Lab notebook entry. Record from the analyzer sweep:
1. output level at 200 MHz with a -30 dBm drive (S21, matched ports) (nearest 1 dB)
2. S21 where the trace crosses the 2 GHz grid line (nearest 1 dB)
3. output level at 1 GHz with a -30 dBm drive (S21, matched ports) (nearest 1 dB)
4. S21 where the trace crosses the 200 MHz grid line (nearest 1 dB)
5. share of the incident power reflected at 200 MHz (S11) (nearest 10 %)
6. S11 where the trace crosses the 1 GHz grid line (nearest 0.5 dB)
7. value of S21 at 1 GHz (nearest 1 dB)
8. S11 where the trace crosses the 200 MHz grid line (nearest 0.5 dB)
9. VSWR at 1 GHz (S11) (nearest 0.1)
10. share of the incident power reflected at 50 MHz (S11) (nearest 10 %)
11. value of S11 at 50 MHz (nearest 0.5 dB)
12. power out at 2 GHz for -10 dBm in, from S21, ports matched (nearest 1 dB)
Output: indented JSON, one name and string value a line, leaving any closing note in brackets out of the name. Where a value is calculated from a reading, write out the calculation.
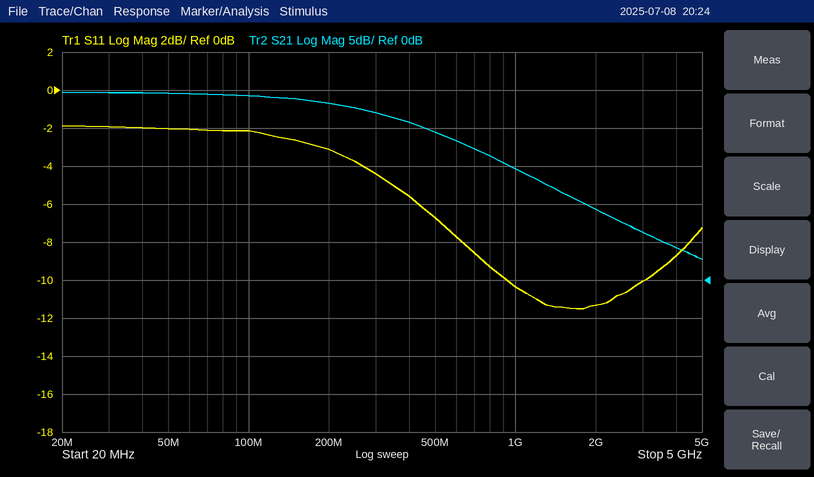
{
  "output level at 200 MHz with a -30 dBm drive (S21, matched ports)": "-30 dBm + (23 dB) = -7 dBm",
  "S21 where the trace crosses the 2 GHz grid line": "9 dB",
  "output level at 1 GHz with a -30 dBm drive (S21, matched ports)": "-30 dBm + (15 dB) = -15 dBm",
  "S21 where the trace crosses the 200 MHz grid line": "23 dB",
  "share of the incident power reflected at 200 MHz (S11)": "10^(-3/10) ≈ 50 %",
  "S11 where the trace crosses the 1 GHz grid line": "-10.5 dB",
  "value of S21 at 1 GHz": "15 dB",
  "S11 where the trace crosses the 200 MHz grid line": "-3.0 dB",
  "VSWR at 1 GHz (S11)": "|Γ| = 10^(-10.5/20) = 0.2985; VSWR = (1 + 0.2985)/(1 − 0.2985) ≈ 1.9",
  "share of the incident power reflected at 50 MHz (S11)": "10^(-2/10) ≈ 63.1 %, so 60 % to the nearest 10 %",
  "value of S11 at 50 MHz": "-2.0 dB",
  "power out at 2 GHz for -10 dBm in, from S21, ports matched": "-10 dBm + (9 dB) = -1 dBm"
}
